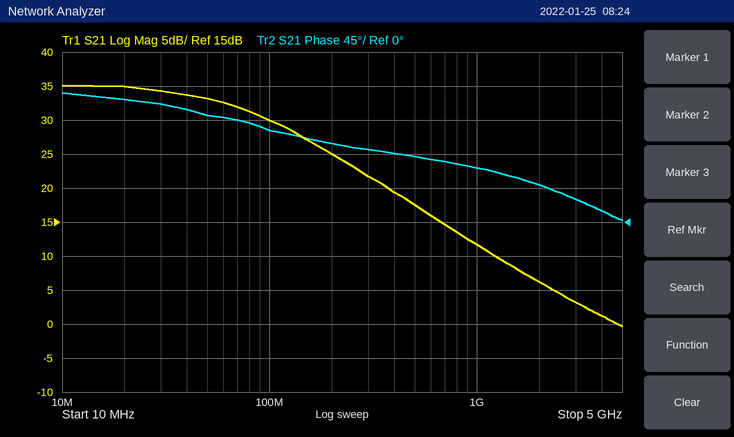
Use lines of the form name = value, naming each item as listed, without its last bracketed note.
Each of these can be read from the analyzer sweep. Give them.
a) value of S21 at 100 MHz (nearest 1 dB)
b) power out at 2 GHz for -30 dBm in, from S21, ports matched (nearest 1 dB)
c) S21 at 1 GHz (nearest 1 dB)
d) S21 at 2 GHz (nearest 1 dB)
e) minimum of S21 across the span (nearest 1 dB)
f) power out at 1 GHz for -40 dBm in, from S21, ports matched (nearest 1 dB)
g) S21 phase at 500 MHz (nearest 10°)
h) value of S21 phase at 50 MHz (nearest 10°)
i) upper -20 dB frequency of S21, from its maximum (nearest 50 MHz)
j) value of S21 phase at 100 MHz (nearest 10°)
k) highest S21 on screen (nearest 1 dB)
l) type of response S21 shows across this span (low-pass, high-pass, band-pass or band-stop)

value of S21 at 100 MHz = 30 dB
power out at 2 GHz for -30 dBm in, from S21, ports matched = -24 dBm
S21 at 1 GHz = 12 dB
S21 at 2 GHz = 6 dB
minimum of S21 across the span = 0 dB
power out at 1 GHz for -40 dBm in, from S21, ports matched = -28 dBm
S21 phase at 500 MHz = 90°
value of S21 phase at 50 MHz = 140°
upper -20 dB frequency of S21, from its maximum = 650 MHz
value of S21 phase at 100 MHz = 120°
highest S21 on screen = 35 dB
type of response S21 shows across this span = low-pass
